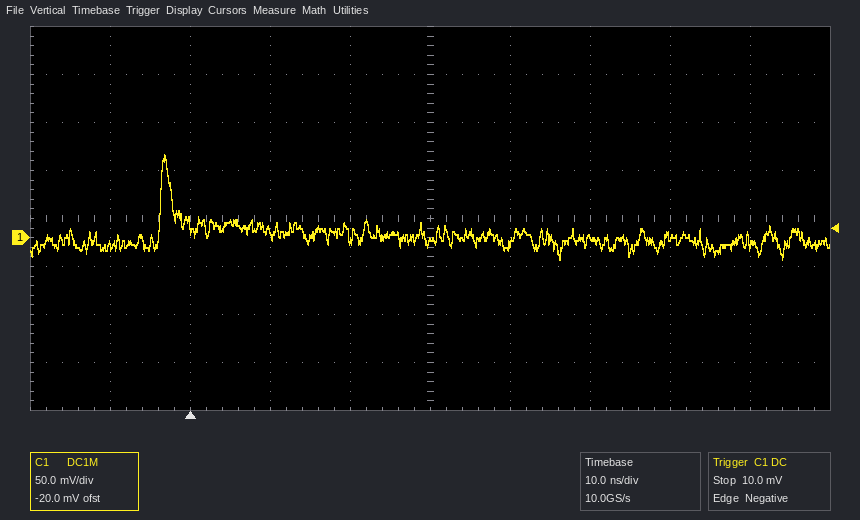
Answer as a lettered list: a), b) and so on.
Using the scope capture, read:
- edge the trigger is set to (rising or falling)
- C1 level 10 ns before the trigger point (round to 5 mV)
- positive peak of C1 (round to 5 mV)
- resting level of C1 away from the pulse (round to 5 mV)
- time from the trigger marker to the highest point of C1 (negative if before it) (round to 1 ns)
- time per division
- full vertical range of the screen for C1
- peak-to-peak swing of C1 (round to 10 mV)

a) falling
b) -10 mV
c) 85 mV
d) 0 mV
e) -3 ns
f) 10 ns
g) 400 mV
h) 110 mV
